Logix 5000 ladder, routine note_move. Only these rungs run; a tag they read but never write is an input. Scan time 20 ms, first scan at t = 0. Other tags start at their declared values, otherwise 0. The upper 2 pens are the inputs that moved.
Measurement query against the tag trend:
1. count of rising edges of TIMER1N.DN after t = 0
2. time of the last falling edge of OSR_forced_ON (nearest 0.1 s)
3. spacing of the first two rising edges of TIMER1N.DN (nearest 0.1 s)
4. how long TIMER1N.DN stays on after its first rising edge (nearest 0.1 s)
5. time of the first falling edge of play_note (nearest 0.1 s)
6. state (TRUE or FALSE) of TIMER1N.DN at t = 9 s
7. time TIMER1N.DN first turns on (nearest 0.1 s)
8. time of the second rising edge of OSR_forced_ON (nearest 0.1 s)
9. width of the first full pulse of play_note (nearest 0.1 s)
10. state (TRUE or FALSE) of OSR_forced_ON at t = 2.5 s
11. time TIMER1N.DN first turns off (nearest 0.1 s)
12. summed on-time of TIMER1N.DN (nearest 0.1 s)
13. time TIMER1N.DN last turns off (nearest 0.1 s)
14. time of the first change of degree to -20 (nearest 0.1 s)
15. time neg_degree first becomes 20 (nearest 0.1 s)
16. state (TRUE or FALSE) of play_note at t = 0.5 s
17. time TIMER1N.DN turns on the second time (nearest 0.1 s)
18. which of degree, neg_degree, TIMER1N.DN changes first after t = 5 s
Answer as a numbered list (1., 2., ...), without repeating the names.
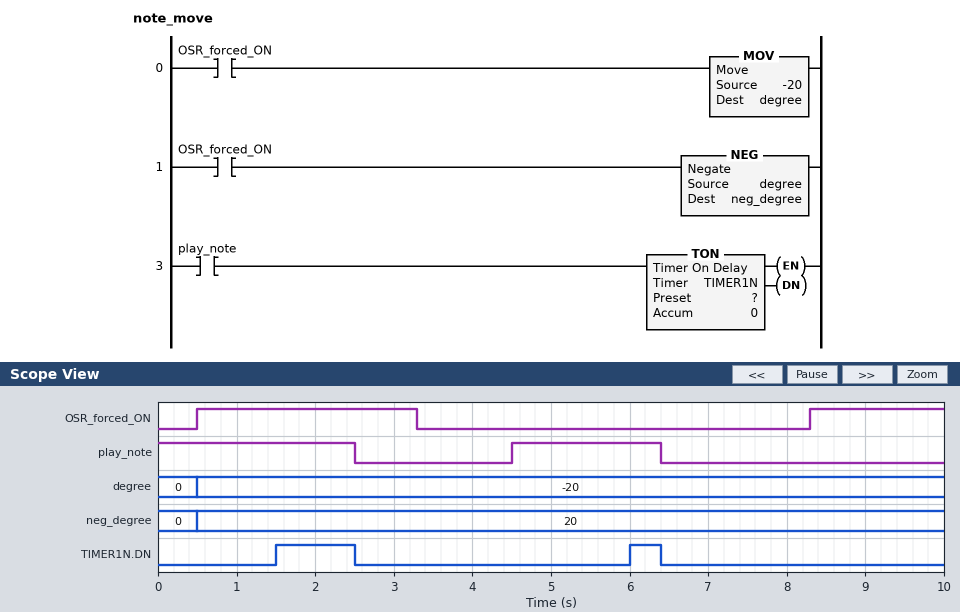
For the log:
1. 2
2. 3.3 s
3. 4.5 s
4. 1.0 s
5. 2.5 s
6. FALSE
7. 1.5 s
8. 8.3 s
9. 1.9 s
10. TRUE
11. 2.5 s
12. 1.4 s
13. 6.4 s
14. 0.5 s
15. 0.5 s
16. TRUE
17. 6.0 s
18. TIMER1N.DN
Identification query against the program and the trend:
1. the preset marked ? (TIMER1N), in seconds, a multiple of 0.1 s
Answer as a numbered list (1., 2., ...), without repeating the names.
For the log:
1. 1.5 s
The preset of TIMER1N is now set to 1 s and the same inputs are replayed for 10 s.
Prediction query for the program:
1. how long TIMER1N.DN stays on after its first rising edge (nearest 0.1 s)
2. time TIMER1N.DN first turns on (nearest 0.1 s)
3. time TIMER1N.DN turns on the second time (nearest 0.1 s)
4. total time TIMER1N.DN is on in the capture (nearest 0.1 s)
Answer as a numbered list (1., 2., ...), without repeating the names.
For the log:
1. 1.5 s
2. 1.0 s
3. 5.5 s
4. 2.4 s
